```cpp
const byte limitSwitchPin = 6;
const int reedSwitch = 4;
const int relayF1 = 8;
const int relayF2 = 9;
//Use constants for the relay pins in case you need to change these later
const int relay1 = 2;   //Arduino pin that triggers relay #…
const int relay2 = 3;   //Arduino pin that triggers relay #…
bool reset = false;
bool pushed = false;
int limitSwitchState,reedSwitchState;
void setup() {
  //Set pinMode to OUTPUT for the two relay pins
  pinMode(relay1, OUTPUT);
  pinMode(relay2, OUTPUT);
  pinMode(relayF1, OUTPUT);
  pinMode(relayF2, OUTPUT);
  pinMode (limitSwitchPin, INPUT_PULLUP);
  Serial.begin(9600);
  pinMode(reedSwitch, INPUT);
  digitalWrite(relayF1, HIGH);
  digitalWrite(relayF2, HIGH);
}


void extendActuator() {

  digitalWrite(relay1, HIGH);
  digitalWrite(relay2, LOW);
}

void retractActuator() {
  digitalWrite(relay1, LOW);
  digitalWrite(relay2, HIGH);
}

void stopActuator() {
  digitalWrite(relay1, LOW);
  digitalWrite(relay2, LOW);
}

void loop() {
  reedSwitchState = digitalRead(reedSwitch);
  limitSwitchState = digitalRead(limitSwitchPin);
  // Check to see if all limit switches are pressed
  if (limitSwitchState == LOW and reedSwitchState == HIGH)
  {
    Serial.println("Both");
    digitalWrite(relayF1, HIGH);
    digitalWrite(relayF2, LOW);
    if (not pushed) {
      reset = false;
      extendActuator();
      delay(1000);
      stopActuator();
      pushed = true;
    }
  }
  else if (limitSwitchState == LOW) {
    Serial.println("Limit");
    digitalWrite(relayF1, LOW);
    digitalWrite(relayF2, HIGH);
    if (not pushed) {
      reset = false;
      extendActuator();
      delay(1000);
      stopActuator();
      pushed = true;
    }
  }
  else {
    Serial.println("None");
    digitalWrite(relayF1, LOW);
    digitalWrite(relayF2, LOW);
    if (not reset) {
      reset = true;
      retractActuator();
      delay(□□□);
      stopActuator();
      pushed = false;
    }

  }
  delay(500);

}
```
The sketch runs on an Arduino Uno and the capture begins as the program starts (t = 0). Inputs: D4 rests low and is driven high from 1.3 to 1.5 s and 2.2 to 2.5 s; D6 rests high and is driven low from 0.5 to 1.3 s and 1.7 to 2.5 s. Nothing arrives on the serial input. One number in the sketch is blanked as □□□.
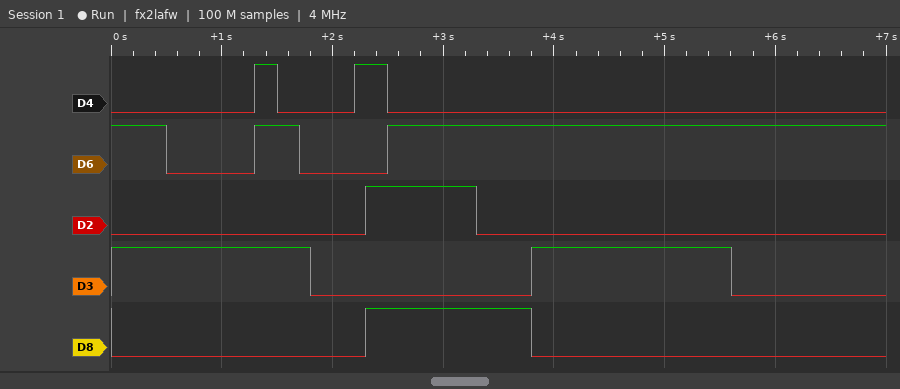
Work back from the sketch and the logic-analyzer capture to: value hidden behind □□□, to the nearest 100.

1800
